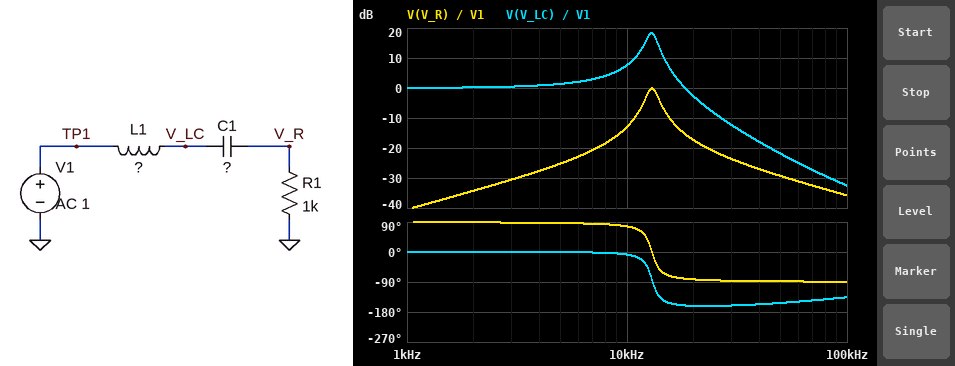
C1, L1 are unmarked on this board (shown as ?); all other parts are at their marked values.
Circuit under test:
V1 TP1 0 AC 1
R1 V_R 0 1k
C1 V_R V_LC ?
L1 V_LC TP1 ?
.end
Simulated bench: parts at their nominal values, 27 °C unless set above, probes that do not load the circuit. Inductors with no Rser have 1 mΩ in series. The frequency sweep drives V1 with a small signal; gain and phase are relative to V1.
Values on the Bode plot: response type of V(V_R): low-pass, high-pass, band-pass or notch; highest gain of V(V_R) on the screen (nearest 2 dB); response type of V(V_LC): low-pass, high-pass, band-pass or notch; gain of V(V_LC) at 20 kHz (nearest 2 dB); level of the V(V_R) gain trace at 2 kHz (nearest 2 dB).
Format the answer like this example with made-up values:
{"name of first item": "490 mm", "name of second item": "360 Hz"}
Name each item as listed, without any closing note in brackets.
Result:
{"response type of V(V_R): low-pass, high-pass, band-pass or notch": "band-pass", "highest gain of V(V_R) on the screen": "0 dB", "response type of V(V_LC): low-pass, high-pass, band-pass or notch": "low-pass", "gain of V(V_LC) at 20 kHz": "-2 dB", "level of the V(V_R) gain trace at 2 kHz": "-34 dB"}
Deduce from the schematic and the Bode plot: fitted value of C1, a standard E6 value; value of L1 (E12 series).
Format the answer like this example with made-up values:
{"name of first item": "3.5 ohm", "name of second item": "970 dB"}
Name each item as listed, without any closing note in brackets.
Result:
{"fitted value of C1, a standard E6 value": "1.5 nF", "value of L1": "100 mH"}
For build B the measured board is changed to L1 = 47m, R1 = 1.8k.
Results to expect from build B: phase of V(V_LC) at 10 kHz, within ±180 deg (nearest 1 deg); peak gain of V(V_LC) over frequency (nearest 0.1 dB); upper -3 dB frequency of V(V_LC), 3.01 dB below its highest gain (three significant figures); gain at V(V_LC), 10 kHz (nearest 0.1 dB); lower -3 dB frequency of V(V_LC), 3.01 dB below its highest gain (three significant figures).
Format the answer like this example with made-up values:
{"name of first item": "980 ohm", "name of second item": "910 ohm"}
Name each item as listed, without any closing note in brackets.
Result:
{"phase of V(V_LC) at 10 kHz, within ±180 deg": "-4 deg", "peak gain of V(V_LC) over frequency": "10.4 dB", "upper -3 dB frequency of V(V_LC), 3.01 dB below its highest gain": "21.4 kHz", "gain at V(V_LC), 10 kHz": "2.7 dB", "lower -3 dB frequency of V(V_LC), 3.01 dB below its highest gain": "15.2 kHz"}
